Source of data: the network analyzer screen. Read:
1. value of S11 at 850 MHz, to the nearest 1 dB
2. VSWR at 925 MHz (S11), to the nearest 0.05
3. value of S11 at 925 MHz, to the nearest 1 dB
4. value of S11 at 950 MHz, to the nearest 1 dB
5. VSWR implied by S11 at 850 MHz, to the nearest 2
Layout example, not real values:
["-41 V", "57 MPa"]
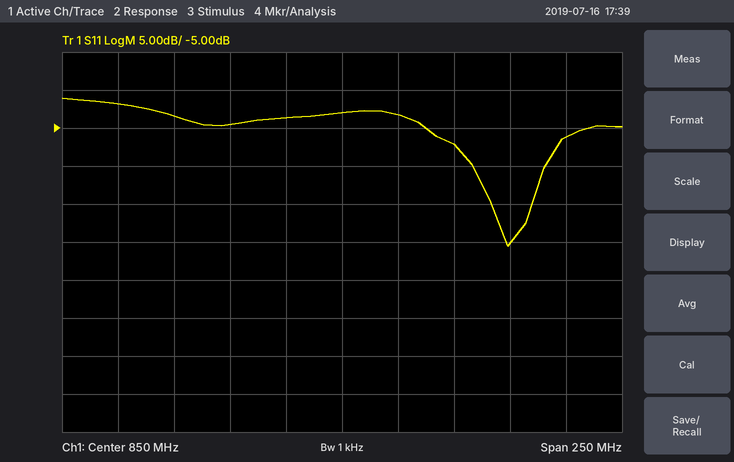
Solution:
["-3 dB", "1.20", "-20 dB", "-6 dB", "6"]
